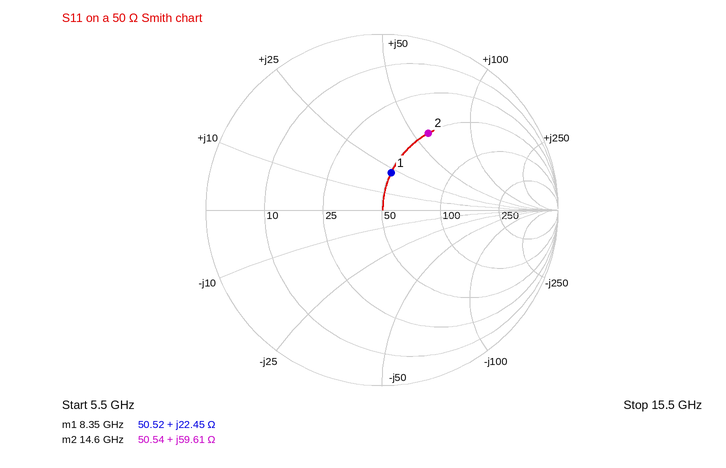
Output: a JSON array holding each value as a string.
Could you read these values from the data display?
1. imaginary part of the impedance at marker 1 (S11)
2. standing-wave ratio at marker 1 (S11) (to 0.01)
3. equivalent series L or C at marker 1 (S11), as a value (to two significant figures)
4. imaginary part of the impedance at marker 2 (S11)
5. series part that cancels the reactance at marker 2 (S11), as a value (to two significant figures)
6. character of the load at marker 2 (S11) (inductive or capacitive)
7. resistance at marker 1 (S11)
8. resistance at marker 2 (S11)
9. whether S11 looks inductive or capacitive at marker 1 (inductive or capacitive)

["+22.45 Ω", "1.56", "430 pH", "+59.61 Ω", "180 fF", "inductive", "50.52 Ω", "50.54 Ω", "inductive"]
